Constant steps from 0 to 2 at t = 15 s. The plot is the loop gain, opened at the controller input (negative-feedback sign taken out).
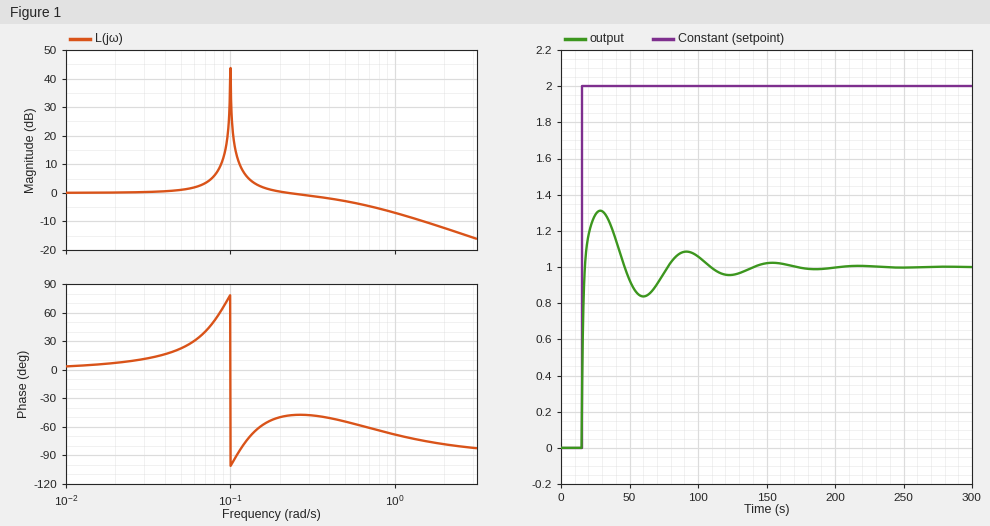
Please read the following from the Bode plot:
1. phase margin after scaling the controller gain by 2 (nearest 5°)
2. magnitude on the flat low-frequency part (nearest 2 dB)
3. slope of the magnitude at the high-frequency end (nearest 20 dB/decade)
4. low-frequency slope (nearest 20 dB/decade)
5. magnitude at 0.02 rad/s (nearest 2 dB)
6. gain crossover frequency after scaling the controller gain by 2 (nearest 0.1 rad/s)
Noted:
115°
0 dB
-20 dB/decade
0 dB/decade
0 dB
0.9 rad/s
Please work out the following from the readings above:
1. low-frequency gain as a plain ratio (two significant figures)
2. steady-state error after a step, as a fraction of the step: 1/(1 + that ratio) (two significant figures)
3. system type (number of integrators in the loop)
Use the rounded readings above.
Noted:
1.0
0.50
0
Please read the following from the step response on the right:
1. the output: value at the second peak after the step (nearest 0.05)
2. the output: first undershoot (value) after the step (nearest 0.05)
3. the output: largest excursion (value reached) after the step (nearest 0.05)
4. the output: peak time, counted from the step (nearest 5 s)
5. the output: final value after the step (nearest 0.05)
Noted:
1.10
0.85
1.30
15 s
1.00
